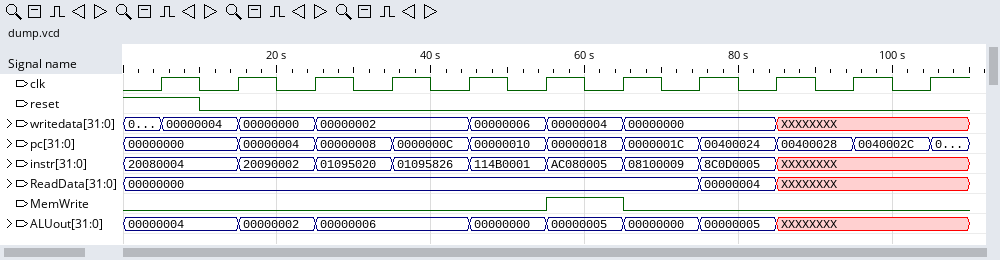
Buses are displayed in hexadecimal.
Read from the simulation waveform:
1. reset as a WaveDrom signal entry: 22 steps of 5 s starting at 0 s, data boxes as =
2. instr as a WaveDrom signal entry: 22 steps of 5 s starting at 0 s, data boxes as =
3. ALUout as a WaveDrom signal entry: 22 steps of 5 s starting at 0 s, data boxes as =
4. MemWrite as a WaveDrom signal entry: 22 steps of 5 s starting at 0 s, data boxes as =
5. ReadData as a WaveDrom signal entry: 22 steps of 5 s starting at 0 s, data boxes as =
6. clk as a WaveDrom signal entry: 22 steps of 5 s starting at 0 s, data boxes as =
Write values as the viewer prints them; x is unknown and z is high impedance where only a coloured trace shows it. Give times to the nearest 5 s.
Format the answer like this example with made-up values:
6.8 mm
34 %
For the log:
{name: 'reset', wave: '1.0...................'}
{name: 'instr', wave: '=..=.=.=.=.=.=.=.x....', data: '20080004 20090002 01095020 01095826 114B0001 AC080005 08100009 8C0D0005'}
{name: 'ALUout', wave: '=..=.=...=.=.=.=.x....', data: '00000004 00000002 00000006 00000000 00000005 00000000 00000005'}
{name: 'MemWrite', wave: '0..........1.0........'}
{name: 'ReadData', wave: '=..............=.x....', data: '00000000 00000004'}
{name: 'clk', wave: '0101010101010101010101'}
